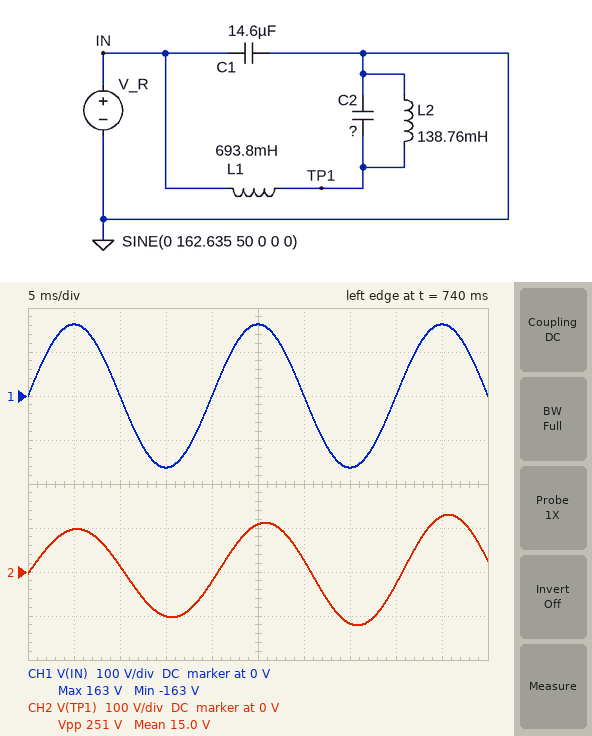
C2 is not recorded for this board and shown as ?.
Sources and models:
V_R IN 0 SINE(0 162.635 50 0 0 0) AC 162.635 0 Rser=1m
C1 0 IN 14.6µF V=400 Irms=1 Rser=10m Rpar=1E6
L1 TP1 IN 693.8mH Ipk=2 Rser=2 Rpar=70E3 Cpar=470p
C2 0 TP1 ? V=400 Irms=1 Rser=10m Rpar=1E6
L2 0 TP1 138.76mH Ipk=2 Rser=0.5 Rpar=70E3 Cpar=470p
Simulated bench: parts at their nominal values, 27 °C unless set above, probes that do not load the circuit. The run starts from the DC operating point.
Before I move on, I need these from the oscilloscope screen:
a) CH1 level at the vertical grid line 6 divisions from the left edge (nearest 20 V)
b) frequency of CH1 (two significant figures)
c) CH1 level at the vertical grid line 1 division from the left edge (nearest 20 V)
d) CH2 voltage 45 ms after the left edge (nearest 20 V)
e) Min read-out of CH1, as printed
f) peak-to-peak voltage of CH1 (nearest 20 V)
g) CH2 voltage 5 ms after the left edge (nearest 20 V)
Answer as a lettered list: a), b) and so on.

a) 0 V
b) 50 Hz
c) 160 V
d) 120 V
e) -163 V
f) 320 V
g) 100 V
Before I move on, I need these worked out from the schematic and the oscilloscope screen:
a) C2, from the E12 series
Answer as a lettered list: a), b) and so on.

a) 68 µF
